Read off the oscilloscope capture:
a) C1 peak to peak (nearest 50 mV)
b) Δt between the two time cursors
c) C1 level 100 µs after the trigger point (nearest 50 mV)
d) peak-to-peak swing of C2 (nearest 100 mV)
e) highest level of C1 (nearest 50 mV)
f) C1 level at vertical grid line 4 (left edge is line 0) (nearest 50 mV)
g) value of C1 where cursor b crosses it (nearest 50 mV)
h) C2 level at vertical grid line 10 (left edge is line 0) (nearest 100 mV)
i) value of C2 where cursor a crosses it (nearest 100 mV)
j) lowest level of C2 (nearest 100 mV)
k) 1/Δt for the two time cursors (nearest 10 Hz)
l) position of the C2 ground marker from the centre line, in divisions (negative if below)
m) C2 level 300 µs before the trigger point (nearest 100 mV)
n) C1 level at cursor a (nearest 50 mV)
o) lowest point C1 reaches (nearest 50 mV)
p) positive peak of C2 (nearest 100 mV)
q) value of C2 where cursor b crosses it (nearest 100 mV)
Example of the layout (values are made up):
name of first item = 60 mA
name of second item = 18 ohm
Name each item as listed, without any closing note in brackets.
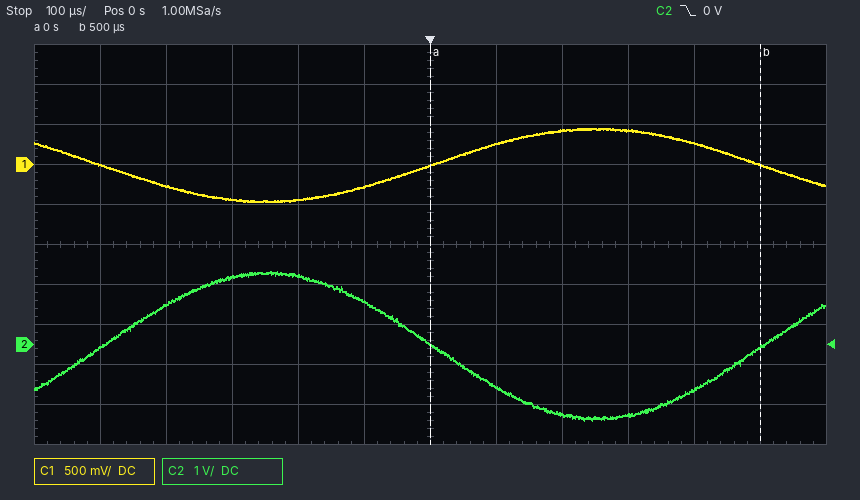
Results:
C1 peak to peak = 900 mV
Δt between the two time cursors = 500 µs
C1 level 100 µs after the trigger point = 250 mV
peak-to-peak swing of C2 = 3.7 V
highest level of C1 = 450 mV
C1 level at vertical grid line 4 (left edge is line 0) = -450 mV
value of C1 where cursor b crosses it = 0 mV
C2 level at vertical grid line 10 (left edge is line 0) = -1.1 V
value of C2 where cursor a crosses it = 0.0 V
lowest level of C2 = -1.9 V
1/Δt for the two time cursors = 2.00 kHz
position of the C2 ground marker from the centre line, in divisions = -2.5 div
C2 level 300 µs before the trigger point = 1.7 V
C1 level at cursor a = 0 mV
lowest point C1 reaches = -450 mV
positive peak of C2 = 1.8 V
value of C2 where cursor b crosses it = -100 mV
